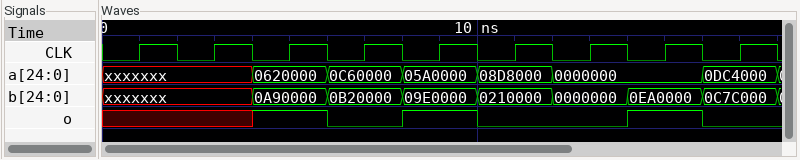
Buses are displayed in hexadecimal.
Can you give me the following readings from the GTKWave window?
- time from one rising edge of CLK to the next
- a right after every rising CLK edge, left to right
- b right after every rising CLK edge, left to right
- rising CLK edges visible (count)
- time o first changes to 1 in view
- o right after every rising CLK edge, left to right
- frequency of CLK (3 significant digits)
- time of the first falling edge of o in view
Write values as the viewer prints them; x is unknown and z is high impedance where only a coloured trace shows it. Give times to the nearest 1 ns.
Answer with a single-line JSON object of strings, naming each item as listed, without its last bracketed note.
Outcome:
{"time from one rising edge of CLK to the next": "2 ns", "a right after every rising CLK edge, left to right": "xxxxxxx, xxxxxxx, 0620000, 0C60000, 05A0000, 08D8000, 0000000, 0000000, 0DC4000", "b right after every rising CLK edge, left to right": "xxxxxxx, xxxxxxx, 0A90000, 0B20000, 09E0000, 0210000, 0000000, 0EA0000, 0C7C000", "rising CLK edges visible": "9", "time o first changes to 1 in view": "4 ns", "o right after every rising CLK edge, left to right": "x x 1 0 1 0 0 1 0", "frequency of CLK": "500 MHz", "time of the first falling edge of o in view": "6 ns"}
